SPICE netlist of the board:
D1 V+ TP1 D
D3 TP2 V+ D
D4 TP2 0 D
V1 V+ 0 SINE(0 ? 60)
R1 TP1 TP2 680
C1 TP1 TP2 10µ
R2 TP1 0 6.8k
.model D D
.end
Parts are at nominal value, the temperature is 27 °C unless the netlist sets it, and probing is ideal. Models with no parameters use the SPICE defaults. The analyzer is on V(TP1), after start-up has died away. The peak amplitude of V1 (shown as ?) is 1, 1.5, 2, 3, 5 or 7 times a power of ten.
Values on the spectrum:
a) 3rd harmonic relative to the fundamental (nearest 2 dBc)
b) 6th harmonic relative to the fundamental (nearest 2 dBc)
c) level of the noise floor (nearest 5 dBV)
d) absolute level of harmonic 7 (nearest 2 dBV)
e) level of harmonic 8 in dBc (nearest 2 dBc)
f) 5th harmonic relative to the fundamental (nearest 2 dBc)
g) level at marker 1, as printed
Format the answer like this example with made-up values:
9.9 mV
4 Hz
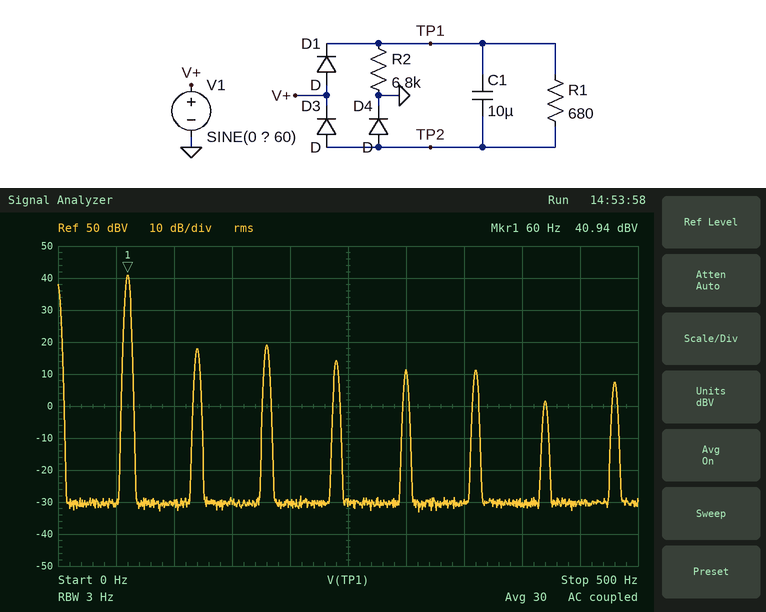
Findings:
-22 dBc
-30 dBc
-30 dBV
2 dBV
-34 dBc
-30 dBc
40.94 dBV
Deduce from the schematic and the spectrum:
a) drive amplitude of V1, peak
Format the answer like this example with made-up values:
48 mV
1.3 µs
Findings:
200 V
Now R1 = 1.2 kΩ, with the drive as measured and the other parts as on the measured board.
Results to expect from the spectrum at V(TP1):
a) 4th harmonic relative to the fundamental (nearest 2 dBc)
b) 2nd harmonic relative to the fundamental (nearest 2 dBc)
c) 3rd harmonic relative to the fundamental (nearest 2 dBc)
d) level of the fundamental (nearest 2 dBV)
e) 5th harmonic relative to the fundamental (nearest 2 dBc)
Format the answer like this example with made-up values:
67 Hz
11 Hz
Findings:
-22 dBc
-18 dBc
-20 dBc
40 dBV
-36 dBc
